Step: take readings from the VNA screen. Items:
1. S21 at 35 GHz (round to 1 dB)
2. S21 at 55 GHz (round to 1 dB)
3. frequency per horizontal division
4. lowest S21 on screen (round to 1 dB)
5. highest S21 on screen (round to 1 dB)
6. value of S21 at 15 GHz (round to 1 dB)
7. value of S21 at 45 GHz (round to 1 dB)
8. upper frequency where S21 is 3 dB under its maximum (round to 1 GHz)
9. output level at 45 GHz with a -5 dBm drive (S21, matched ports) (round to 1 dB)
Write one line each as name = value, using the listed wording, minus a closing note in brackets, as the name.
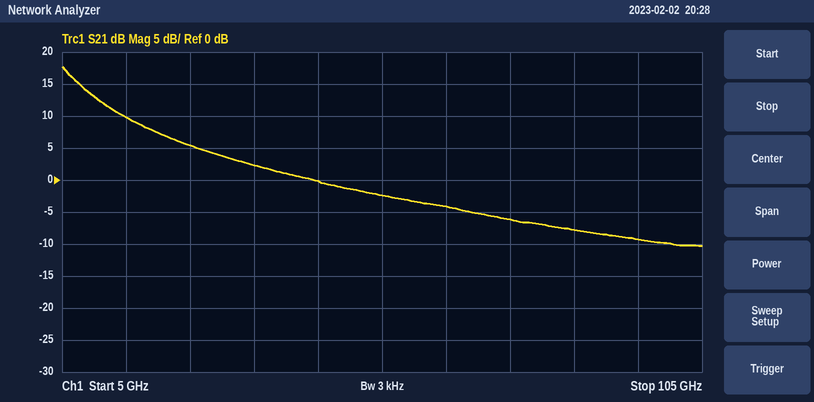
S21 at 35 GHz = 2 dB
S21 at 55 GHz = -2 dB
frequency per horizontal division = 10 GHz
lowest S21 on screen = -10 dB
highest S21 on screen = 18 dB
value of S21 at 15 GHz = 10 dB
value of S21 at 45 GHz = 0 dB
upper frequency where S21 is 3 dB under its maximum = 8 GHz
output level at 45 GHz with a -5 dBm drive (S21, matched ports) = -5 dBm
